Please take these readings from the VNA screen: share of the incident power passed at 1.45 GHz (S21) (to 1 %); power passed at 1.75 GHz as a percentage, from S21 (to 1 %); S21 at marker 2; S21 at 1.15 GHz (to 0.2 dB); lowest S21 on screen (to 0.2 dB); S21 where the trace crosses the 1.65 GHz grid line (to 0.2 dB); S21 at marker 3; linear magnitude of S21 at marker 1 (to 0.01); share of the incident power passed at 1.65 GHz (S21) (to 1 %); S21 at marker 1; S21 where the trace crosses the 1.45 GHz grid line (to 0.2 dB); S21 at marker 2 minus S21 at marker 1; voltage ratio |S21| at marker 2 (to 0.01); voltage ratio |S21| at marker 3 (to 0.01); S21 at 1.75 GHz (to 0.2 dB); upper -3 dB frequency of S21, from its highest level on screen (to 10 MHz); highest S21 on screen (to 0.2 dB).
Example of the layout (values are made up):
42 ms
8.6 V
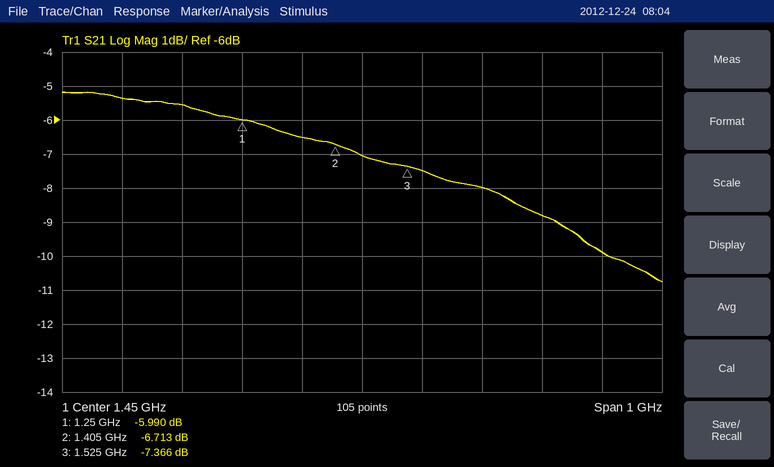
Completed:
20 %
13 %
-6.713 dB
-5.6 dB
-10.8 dB
-8.0 dB
-7.366 dB
0.50
16 %
-5.990 dB
-7.0 dB
-0.723 dB
0.46
0.43
-8.8 dB
1.68 GHz
-5.2 dB
